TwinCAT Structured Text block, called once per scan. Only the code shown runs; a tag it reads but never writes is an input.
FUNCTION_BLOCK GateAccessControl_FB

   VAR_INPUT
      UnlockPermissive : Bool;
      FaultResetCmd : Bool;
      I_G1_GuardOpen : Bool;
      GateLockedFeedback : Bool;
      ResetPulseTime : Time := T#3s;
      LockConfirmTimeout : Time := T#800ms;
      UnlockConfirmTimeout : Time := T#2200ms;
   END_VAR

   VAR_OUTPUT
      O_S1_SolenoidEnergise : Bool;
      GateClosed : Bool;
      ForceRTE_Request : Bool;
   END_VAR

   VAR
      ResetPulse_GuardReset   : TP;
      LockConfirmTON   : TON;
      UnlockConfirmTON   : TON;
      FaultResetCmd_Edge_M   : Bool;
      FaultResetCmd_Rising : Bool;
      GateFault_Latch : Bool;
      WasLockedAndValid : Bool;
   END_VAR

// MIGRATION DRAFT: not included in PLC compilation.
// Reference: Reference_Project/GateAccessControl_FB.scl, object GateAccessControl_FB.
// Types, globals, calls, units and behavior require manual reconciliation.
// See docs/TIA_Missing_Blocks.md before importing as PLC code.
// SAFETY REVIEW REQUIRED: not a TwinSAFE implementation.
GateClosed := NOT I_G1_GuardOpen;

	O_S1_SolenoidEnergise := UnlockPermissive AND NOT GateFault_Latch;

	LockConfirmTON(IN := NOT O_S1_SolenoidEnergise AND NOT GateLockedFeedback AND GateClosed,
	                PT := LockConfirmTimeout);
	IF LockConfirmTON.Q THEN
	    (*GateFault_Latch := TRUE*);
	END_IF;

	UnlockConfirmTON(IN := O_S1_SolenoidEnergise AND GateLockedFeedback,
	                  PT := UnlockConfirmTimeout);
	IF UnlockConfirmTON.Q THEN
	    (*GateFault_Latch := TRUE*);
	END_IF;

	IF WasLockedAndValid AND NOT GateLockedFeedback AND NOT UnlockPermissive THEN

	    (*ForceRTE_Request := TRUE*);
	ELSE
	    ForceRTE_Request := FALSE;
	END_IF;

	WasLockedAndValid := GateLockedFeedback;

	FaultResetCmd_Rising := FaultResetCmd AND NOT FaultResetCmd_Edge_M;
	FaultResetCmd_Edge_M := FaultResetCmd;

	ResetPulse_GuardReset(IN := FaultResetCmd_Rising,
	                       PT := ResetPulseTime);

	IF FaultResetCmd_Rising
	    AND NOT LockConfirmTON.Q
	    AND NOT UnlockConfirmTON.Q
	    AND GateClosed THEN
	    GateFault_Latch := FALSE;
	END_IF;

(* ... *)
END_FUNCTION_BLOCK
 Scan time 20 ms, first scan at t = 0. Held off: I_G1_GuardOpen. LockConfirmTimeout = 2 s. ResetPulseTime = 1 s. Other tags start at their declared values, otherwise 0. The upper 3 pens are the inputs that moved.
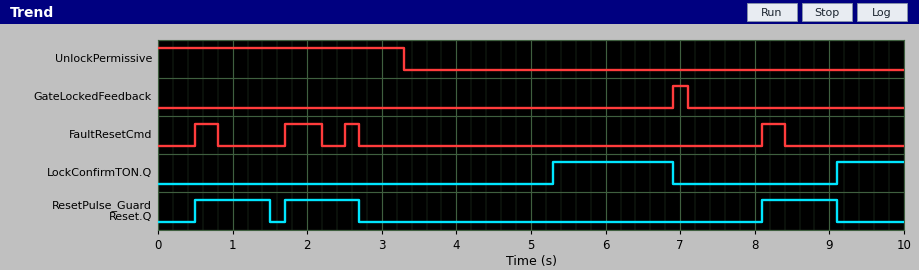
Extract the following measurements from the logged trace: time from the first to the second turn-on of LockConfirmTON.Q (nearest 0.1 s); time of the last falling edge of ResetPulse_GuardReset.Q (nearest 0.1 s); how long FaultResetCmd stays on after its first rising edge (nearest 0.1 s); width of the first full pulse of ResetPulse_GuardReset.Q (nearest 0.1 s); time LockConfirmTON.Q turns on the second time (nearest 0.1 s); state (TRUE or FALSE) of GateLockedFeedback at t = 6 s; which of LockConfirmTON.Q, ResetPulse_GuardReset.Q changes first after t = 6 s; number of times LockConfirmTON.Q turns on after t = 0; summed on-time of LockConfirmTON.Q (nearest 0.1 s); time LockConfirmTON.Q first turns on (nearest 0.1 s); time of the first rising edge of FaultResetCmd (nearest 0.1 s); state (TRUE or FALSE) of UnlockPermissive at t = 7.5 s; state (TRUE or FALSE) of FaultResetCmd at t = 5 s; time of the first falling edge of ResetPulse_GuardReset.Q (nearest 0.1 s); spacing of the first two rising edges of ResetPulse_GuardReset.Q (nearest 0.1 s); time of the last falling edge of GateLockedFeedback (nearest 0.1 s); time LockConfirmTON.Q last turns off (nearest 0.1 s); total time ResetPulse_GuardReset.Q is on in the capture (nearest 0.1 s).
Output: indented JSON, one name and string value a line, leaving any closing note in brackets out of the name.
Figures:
{
  "time from the first to the second turn-on of LockConfirmTON.Q": "3.8 s",
  "time of the last falling edge of ResetPulse_GuardReset.Q": "9.1 s",
  "how long FaultResetCmd stays on after its first rising edge": "0.3 s",
  "width of the first full pulse of ResetPulse_GuardReset.Q": "1.0 s",
  "time LockConfirmTON.Q turns on the second time": "9.1 s",
  "state (TRUE or FALSE) of GateLockedFeedback at t = 6 s": "FALSE",
  "which of LockConfirmTON.Q, ResetPulse_GuardReset.Q changes first after t = 6 s": "LockConfirmTON.Q",
  "number of times LockConfirmTON.Q turns on after t = 0": "2",
  "summed on-time of LockConfirmTON.Q": "2.5 s",
  "time LockConfirmTON.Q first turns on": "5.3 s",
  "time of the first rising edge of FaultResetCmd": "0.5 s",
  "state (TRUE or FALSE) of UnlockPermissive at t = 7.5 s": "FALSE",
  "state (TRUE or FALSE) of FaultResetCmd at t = 5 s": "FALSE",
  "time of the first falling edge of ResetPulse_GuardReset.Q": "1.5 s",
  "spacing of the first two rising edges of ResetPulse_GuardReset.Q": "1.2 s",
  "time of the last falling edge of GateLockedFeedback": "7.1 s",
  "time LockConfirmTON.Q last turns off": "6.9 s",
  "total time ResetPulse_GuardReset.Q is on in the capture": "3.0 s"
}
